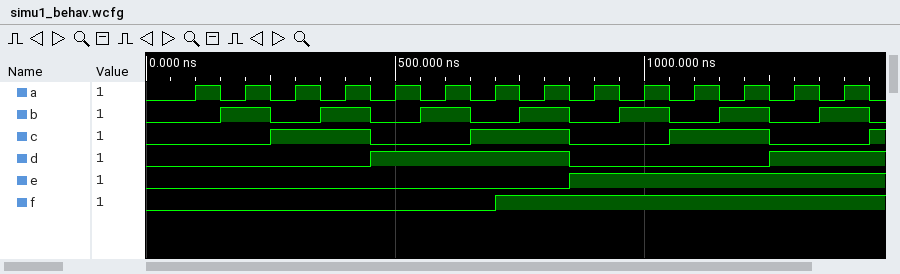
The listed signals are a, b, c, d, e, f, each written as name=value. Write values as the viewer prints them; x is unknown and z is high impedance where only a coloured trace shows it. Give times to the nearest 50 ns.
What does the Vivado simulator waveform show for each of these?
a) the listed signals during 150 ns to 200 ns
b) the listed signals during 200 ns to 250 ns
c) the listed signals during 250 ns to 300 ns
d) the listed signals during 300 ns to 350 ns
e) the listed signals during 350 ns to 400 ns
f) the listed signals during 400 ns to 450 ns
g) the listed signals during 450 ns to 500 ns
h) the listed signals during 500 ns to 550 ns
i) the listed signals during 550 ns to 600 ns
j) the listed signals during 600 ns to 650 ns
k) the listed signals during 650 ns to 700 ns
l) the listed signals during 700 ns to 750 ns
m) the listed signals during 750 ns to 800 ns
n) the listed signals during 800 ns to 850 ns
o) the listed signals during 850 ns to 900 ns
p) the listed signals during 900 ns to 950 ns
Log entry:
a=0, b=1, c=0, d=0, e=0, f=0
a=1, b=1, c=0, d=0, e=0, f=0
a=0, b=0, c=1, d=0, e=0, f=0
a=1, b=0, c=1, d=0, e=0, f=0
a=0, b=1, c=1, d=0, e=0, f=0
a=1, b=1, c=1, d=0, e=0, f=0
a=0, b=0, c=0, d=1, e=0, f=0
a=1, b=0, c=0, d=1, e=0, f=0
a=0, b=1, c=0, d=1, e=0, f=0
a=1, b=1, c=0, d=1, e=0, f=0
a=0, b=0, c=1, d=1, e=0, f=0
a=1, b=0, c=1, d=1, e=0, f=1
a=0, b=1, c=1, d=1, e=0, f=1
a=1, b=1, c=1, d=1, e=0, f=1
a=0, b=0, c=0, d=0, e=1, f=1
a=1, b=0, c=0, d=0, e=1, f=1
